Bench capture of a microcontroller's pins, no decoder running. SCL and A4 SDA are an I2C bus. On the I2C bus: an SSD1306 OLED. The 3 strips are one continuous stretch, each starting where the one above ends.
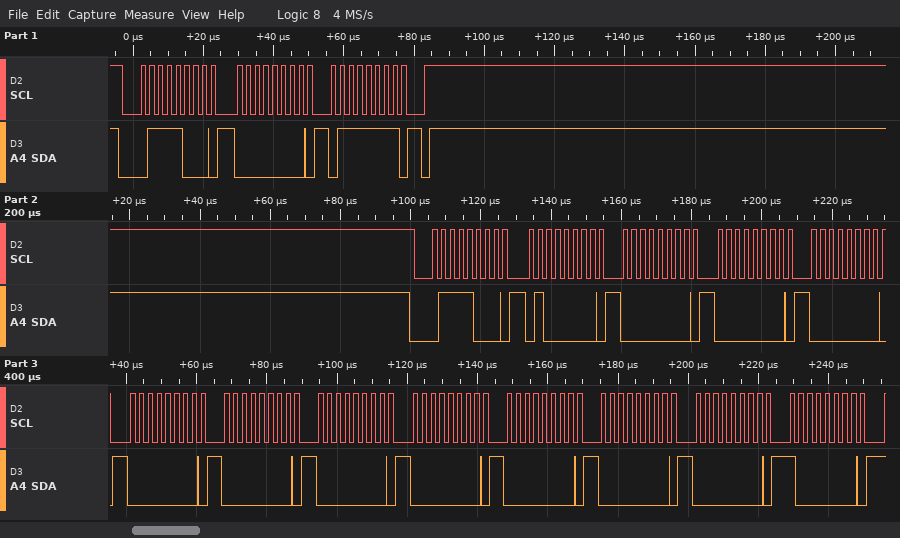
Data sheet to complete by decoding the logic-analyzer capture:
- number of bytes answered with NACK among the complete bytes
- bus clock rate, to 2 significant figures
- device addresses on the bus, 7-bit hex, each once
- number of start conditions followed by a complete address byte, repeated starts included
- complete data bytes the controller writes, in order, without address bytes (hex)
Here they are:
0
400 kHz
0x3C
2
00 7F 40 00 00 00 00 00 00 00 00 00 00 80
